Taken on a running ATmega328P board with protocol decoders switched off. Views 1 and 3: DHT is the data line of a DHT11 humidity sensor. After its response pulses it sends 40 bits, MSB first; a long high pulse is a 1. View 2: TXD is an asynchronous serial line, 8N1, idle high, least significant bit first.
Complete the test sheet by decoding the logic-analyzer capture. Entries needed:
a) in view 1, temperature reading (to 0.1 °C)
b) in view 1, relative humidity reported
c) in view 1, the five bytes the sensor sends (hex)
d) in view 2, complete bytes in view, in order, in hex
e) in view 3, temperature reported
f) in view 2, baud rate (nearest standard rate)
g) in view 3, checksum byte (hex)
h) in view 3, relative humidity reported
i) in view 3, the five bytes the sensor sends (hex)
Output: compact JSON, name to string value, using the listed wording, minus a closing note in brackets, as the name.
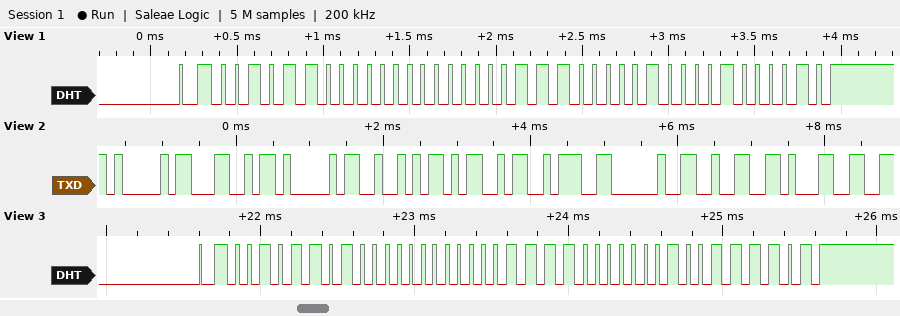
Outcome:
{"in view 1, temperature reading": "14.8 °C", "in view 1, relative humidity reported": "44 %", "in view 1, the five bytes the sensor sends": "2C 00 0E 08 42", "in view 2, complete bytes in view, in order, in hex": "0x41 0x4C 0x41 0x52 0x4D 0x3A 0x20 0x32 0x31", "in view 3, temperature reported": "15.1 °C", "in view 2, baud rate": "9600 baud", "in view 3, checksum byte": "0x3D", "in view 3, relative humidity reported": "45 %", "in view 3, the five bytes the sensor sends": "2D 00 0F 01 3D"}
